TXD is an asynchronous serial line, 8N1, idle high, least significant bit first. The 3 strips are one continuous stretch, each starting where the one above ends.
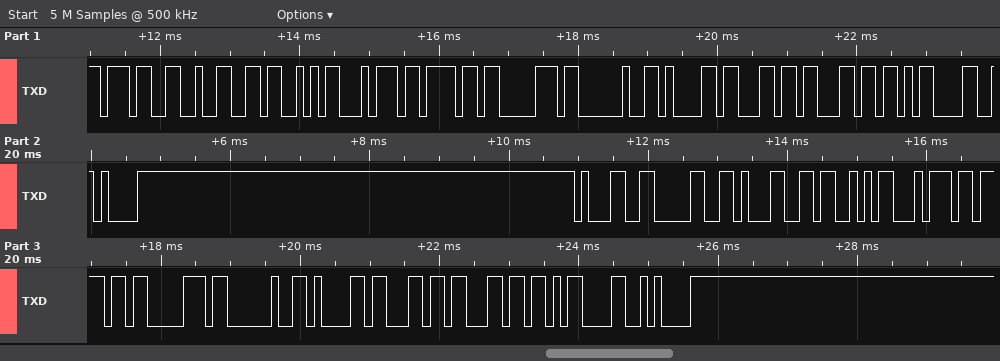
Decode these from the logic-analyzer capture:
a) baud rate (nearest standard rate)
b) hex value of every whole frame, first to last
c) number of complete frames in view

9600 baud
37 32 53 74 6F 70 20 61 6C 6C 0D 0A 31 30 31 53 74 6F 70 20 61 6C 6C 0D 0A
25
